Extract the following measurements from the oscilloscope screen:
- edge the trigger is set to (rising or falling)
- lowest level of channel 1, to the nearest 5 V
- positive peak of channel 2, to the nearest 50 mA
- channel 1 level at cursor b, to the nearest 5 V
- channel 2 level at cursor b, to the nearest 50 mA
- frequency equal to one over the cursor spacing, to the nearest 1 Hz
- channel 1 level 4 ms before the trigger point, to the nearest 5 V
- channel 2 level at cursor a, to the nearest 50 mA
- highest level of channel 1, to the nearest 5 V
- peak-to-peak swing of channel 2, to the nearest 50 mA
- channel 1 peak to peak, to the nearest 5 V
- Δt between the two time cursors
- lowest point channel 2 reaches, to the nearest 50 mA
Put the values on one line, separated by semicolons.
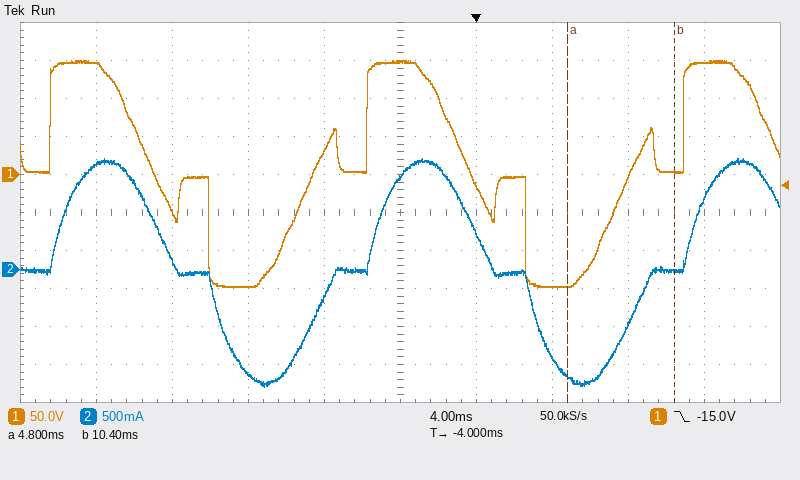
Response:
falling; -150 V; 1.45 A; 5 V; 0 mA; 179 Hz; 150 V; -1.40 A; 150 V; 3.00 A; 300 V; 5.6 ms; -1.55 A
